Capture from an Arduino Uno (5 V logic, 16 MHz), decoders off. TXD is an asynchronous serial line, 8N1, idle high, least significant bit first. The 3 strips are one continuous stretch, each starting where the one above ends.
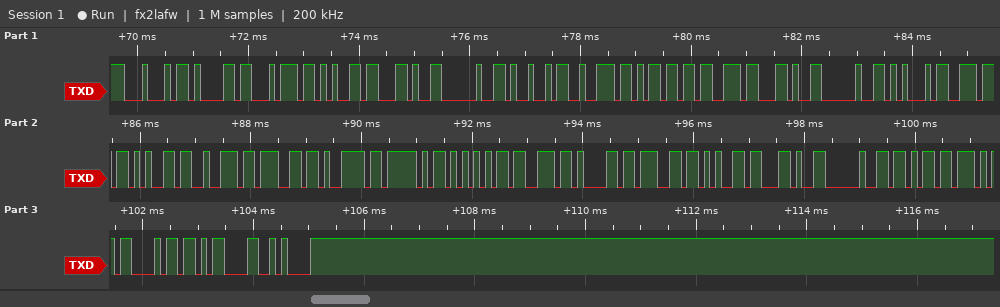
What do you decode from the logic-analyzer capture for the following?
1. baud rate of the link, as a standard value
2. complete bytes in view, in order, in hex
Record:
9600 baud
44 61 74 65 2C 20 49 72 6D 73 2C 20 45 6E 65 72 67 79 5F 55 73 61 67 65 2C 20 6B 57 68 0D 0A
